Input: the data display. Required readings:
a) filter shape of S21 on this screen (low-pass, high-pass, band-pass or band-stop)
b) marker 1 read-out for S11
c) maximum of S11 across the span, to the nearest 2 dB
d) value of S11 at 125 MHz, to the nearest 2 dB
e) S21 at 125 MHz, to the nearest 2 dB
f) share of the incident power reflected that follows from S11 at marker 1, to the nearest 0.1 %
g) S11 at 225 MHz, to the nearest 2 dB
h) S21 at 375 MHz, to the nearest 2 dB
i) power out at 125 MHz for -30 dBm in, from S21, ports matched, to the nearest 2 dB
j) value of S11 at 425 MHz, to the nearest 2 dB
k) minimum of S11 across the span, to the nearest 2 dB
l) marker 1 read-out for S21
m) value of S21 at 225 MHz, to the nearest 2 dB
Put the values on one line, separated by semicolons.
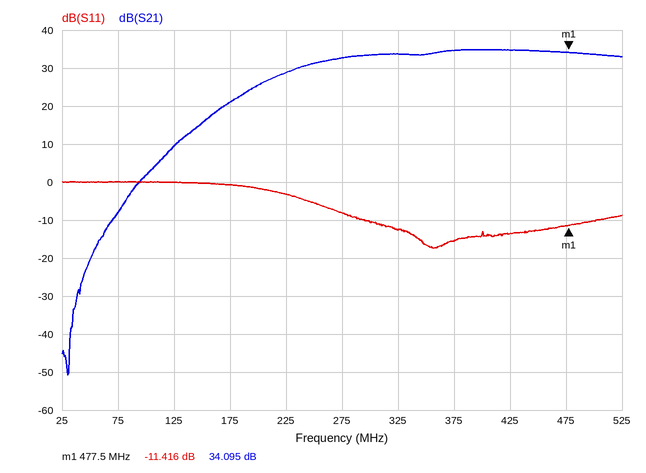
high-pass; -11.416 dB; 0 dB; 0 dB; 10 dB; 7.2 %; -4 dB; 34 dB; -20 dBm; -14 dB; -18 dB; 34.095 dB; 28 dB
